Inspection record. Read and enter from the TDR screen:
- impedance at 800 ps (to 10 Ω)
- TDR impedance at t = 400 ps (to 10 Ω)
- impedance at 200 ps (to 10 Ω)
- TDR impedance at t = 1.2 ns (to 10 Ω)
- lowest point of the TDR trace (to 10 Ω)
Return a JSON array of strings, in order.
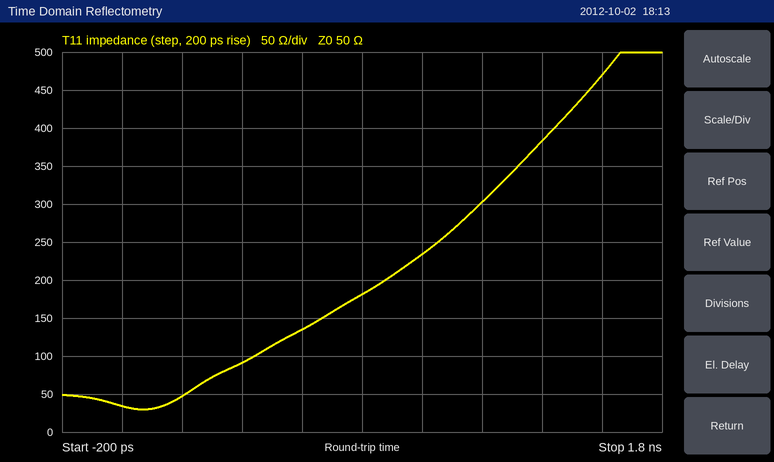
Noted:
["180 Ω", "90 Ω", "50 Ω", "300 Ω", "30 Ω"]
